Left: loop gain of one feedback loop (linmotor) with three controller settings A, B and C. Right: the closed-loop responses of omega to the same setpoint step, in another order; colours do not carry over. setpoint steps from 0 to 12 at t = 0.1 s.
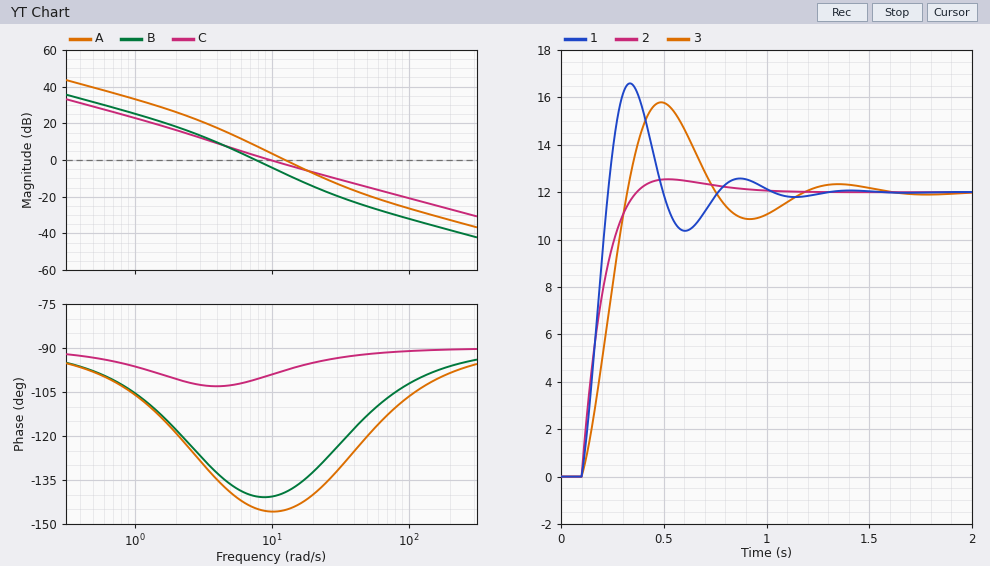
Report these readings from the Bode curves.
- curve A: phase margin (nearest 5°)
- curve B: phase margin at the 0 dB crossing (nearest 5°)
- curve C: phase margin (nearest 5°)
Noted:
35°
40°
80°
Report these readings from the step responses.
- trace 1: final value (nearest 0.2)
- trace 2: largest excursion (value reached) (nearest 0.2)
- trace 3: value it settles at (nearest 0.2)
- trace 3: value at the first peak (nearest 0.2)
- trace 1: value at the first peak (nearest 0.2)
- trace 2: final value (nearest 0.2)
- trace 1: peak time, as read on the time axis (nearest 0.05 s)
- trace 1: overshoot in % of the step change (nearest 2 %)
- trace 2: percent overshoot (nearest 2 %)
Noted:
12.0
12.6
12.0
15.8
16.6
12.0
0.35 s
38 %
4 %
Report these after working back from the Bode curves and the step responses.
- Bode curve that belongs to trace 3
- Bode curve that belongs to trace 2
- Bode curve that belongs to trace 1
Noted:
B
C
A
